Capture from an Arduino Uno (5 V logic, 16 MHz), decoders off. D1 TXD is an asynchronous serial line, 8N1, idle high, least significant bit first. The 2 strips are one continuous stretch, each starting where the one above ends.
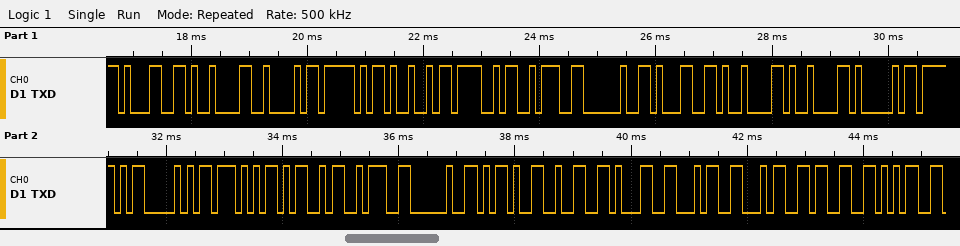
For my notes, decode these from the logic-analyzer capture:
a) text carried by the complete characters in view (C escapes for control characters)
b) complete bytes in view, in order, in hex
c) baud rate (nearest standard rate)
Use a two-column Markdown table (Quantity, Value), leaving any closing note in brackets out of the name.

| Quantity | Value |
|---|---|
| text carried by the complete characters in view | "1\tB_IO: 1\t\tA_PWM: -214435" |
| complete bytes in view, in order, in hex | 31 09 42 5F 49 4F 3A 20 31 09 09 41 5F 50 57 4D 3A 20 2D 32 31 34 34 33 35 |
| baud rate | 9600 baud |
